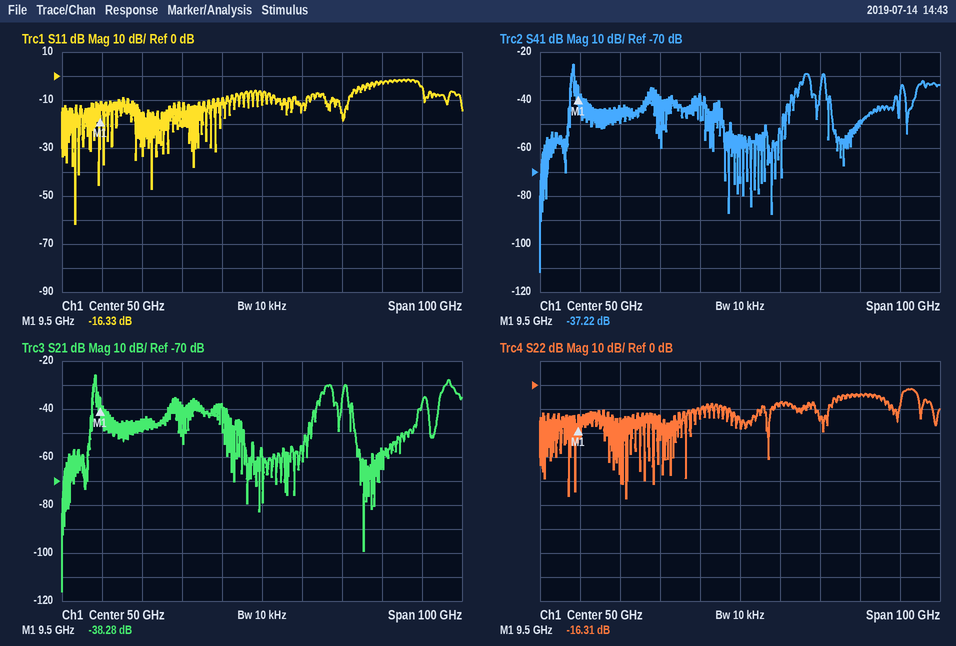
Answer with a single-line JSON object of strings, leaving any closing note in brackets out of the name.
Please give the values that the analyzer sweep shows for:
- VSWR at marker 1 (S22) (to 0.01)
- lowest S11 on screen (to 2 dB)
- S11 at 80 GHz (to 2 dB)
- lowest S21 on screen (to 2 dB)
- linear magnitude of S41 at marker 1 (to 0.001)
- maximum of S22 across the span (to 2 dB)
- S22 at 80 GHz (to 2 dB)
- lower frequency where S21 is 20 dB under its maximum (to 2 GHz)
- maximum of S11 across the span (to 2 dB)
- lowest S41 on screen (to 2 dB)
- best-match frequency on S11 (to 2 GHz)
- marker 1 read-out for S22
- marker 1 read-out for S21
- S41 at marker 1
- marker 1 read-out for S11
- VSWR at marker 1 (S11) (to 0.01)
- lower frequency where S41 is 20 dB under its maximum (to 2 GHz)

{"VSWR at marker 1 (S22)": "1.36", "lowest S11 on screen": "-62 dB", "S11 at 80 GHz": "-2 dB", "lowest S21 on screen": "-116 dB", "linear magnitude of S41 at marker 1": "0.014", "maximum of S22 across the span": "-2 dB", "S22 at 80 GHz": "-4 dB", "lower frequency where S21 is 20 dB under its maximum": "8 GHz", "maximum of S11 across the span": "-2 dB", "lowest S41 on screen": "-112 dB", "best-match frequency on S11": "4 GHz", "marker 1 read-out for S22": "-16.31 dB", "marker 1 read-out for S21": "-38.28 dB", "S41 at marker 1": "-37.22 dB", "marker 1 read-out for S11": "-16.33 dB", "VSWR at marker 1 (S11)": "1.36", "lower frequency where S41 is 20 dB under its maximum": "8 GHz"}
